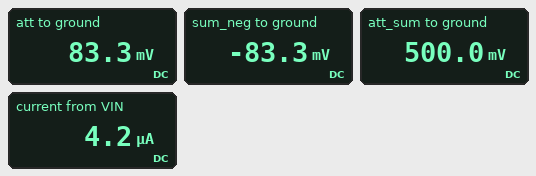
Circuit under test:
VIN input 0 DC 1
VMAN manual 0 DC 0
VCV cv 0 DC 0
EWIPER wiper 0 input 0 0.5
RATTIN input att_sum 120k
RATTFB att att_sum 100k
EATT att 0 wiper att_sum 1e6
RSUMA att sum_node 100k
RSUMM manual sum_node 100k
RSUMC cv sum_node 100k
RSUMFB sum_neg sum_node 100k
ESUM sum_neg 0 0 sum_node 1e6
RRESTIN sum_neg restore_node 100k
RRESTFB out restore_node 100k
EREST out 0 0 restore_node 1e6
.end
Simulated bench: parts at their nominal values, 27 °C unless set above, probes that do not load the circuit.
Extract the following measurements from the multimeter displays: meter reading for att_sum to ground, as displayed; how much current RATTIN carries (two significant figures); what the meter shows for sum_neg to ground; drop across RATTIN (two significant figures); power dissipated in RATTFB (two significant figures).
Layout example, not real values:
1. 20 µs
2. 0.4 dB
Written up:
1. 500.0 mV
2. 4.2 µA
3. -83.3 mV
4. 500 mV
5. 1.7 µW
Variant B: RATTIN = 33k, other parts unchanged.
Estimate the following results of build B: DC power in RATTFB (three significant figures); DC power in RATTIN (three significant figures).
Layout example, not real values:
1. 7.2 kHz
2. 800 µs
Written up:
1. 23.0 µW
2. 7.58 µW
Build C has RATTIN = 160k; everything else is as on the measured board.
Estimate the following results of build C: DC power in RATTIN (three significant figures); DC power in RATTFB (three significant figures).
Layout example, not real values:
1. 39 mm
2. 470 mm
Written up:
1. 1.56 µW
2. 977 nW
